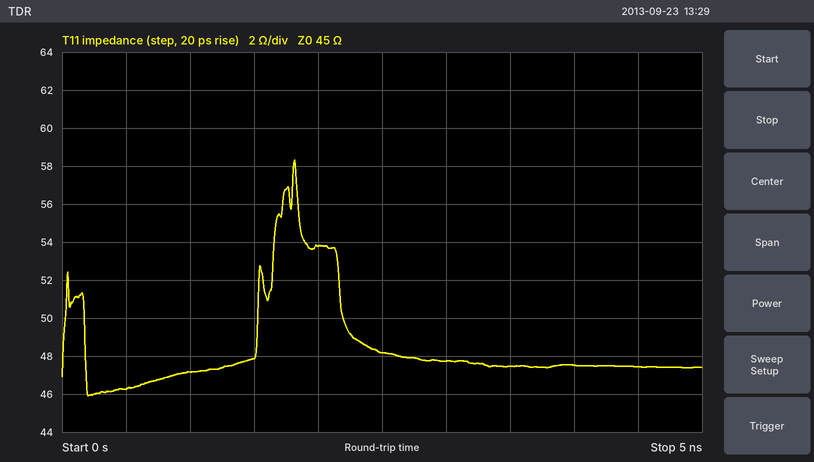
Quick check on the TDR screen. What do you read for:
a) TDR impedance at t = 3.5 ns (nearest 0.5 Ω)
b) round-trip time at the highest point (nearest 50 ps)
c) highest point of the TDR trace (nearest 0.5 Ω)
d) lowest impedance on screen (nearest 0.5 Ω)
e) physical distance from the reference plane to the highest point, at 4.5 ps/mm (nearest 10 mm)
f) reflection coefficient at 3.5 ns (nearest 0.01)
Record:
47.5 Ω
1.80 ns
58.5 Ω
46.0 Ω
200 mm
+0.03
